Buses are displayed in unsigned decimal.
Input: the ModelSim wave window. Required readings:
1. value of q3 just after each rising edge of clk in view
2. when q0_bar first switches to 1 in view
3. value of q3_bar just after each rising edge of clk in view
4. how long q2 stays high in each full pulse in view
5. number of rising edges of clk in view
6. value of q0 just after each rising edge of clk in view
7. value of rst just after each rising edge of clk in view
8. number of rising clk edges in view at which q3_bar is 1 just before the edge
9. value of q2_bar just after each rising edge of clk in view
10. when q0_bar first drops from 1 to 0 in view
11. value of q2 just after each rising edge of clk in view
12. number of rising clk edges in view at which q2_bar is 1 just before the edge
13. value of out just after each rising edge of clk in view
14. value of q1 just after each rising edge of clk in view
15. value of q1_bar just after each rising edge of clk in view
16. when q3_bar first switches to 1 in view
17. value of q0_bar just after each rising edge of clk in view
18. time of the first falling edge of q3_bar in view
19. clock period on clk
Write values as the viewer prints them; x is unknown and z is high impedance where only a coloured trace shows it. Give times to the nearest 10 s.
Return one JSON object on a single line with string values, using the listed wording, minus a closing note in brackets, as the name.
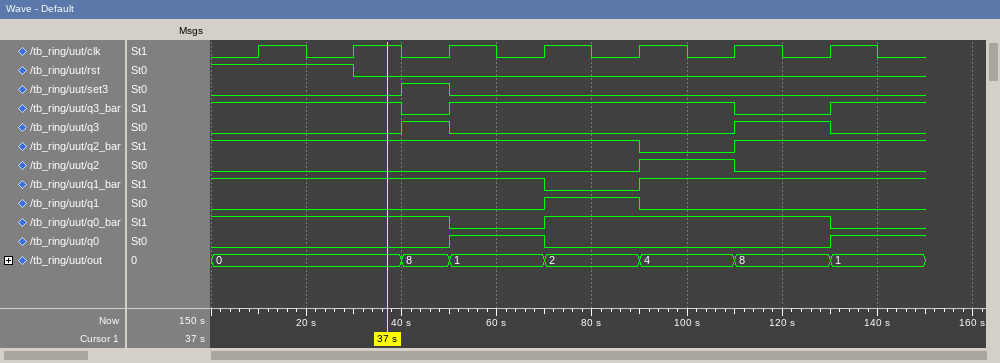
{"value of q3 just after each rising edge of clk in view": "0 0 0 0 0 1 0", "when q0_bar first switches to 1 in view": "70 s", "value of q3_bar just after each rising edge of clk in view": "1 1 1 1 1 0 1", "how long q2 stays high in each full pulse in view": "20 s", "number of rising edges of clk in view": "7", "value of q0 just after each rising edge of clk in view": "0 0 1 0 0 0 1", "value of rst just after each rising edge of clk in view": "1 0 0 0 0 0 0", "number of rising clk edges in view at which q3_bar is 1 just before the edge": "5", "value of q2_bar just after each rising edge of clk in view": "1 1 1 1 0 1 1", "when q0_bar first drops from 1 to 0 in view": "50 s", "value of q2 just after each rising edge of clk in view": "0 0 0 0 1 0 0", "number of rising clk edges in view at which q2_bar is 1 just before the edge": "6", "value of out just after each rising edge of clk in view": "0, 0, 1, 2, 4, 8, 1", "value of q1 just after each rising edge of clk in view": "0 0 0 1 0 0 0", "value of q1_bar just after each rising edge of clk in view": "1 1 1 0 1 1 1", "when q3_bar first switches to 1 in view": "50 s", "value of q0_bar just after each rising edge of clk in view": "1 1 0 1 1 1 0", "time of the first falling edge of q3_bar in view": "40 s", "clock period on clk": "20 s"}
